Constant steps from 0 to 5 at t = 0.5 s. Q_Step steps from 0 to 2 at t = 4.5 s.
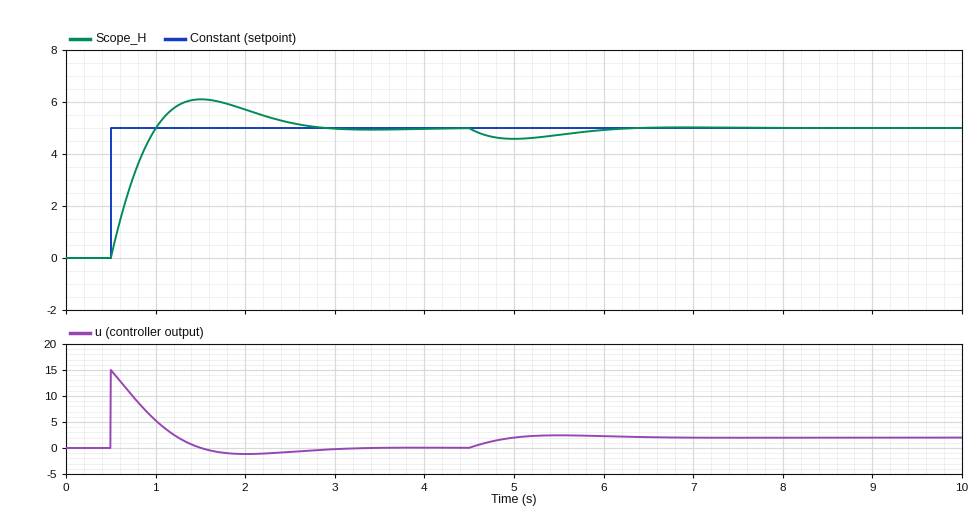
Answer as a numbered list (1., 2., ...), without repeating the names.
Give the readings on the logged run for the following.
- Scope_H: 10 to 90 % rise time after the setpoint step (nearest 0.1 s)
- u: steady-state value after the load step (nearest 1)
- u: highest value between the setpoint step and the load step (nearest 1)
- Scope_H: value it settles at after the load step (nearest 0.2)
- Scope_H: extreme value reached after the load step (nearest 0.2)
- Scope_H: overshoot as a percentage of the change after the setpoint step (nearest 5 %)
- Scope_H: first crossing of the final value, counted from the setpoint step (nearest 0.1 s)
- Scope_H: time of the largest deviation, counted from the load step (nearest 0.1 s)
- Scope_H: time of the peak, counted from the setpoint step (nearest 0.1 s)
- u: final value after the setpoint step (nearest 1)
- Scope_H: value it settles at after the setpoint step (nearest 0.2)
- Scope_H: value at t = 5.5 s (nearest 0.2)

1. 0.4 s
2. 2
3. 15
4. 5.0
5. 4.6
6. 20 %
7. 0.5 s
8. 0.5 s
9. 1.0 s
10. 0
11. 5.0
12. 4.8
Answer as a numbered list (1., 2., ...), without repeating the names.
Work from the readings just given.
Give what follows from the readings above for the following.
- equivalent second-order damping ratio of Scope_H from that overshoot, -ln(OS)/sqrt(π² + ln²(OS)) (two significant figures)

1. 0.46
